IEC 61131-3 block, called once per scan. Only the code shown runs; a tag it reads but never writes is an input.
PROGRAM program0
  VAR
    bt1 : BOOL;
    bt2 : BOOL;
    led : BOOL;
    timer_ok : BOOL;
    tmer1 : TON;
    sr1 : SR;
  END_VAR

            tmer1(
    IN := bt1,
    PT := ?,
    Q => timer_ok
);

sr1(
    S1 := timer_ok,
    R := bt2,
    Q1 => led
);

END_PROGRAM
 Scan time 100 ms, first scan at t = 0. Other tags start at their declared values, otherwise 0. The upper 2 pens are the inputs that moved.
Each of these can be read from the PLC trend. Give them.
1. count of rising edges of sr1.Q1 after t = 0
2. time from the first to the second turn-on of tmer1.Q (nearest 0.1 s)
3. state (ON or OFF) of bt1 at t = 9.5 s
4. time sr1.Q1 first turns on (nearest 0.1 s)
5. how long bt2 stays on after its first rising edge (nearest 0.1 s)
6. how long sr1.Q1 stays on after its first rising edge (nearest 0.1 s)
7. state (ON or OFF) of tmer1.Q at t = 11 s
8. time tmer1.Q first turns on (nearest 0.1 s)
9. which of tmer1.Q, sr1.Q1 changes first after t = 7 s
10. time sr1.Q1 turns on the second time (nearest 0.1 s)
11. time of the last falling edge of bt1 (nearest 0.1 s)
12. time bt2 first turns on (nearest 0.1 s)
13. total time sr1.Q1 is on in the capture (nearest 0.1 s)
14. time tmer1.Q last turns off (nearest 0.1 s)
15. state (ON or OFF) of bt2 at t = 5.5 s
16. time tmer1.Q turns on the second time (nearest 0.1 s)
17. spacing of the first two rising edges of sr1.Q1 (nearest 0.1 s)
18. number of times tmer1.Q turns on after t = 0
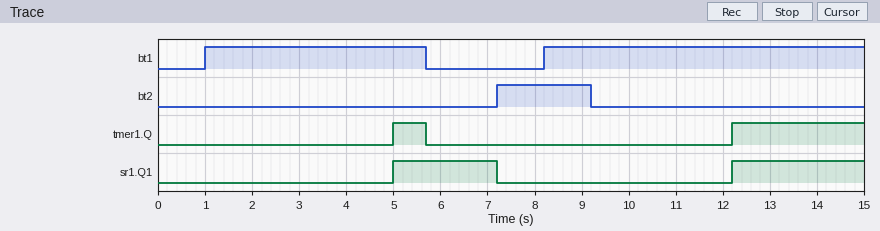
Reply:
2
7.2 s
ON
5.0 s
2.0 s
2.2 s
OFF
5.0 s
sr1.Q1
12.2 s
5.7 s
7.2 s
5.0 s
5.7 s
OFF
12.2 s
7.2 s
2
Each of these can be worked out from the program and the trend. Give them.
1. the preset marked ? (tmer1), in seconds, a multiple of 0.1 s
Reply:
4.0 s
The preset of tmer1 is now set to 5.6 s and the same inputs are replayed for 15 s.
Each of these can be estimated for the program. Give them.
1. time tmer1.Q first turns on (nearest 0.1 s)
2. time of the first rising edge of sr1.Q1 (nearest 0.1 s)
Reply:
13.8 s
13.8 s
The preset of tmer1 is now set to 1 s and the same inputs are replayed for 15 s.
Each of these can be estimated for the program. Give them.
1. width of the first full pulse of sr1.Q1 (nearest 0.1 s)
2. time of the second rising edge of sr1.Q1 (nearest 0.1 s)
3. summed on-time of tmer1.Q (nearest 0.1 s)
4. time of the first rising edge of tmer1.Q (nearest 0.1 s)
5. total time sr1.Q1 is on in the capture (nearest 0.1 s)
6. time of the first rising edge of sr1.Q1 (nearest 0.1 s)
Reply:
5.2 s
9.2 s
9.5 s
2.0 s
11.0 s
2.0 s
